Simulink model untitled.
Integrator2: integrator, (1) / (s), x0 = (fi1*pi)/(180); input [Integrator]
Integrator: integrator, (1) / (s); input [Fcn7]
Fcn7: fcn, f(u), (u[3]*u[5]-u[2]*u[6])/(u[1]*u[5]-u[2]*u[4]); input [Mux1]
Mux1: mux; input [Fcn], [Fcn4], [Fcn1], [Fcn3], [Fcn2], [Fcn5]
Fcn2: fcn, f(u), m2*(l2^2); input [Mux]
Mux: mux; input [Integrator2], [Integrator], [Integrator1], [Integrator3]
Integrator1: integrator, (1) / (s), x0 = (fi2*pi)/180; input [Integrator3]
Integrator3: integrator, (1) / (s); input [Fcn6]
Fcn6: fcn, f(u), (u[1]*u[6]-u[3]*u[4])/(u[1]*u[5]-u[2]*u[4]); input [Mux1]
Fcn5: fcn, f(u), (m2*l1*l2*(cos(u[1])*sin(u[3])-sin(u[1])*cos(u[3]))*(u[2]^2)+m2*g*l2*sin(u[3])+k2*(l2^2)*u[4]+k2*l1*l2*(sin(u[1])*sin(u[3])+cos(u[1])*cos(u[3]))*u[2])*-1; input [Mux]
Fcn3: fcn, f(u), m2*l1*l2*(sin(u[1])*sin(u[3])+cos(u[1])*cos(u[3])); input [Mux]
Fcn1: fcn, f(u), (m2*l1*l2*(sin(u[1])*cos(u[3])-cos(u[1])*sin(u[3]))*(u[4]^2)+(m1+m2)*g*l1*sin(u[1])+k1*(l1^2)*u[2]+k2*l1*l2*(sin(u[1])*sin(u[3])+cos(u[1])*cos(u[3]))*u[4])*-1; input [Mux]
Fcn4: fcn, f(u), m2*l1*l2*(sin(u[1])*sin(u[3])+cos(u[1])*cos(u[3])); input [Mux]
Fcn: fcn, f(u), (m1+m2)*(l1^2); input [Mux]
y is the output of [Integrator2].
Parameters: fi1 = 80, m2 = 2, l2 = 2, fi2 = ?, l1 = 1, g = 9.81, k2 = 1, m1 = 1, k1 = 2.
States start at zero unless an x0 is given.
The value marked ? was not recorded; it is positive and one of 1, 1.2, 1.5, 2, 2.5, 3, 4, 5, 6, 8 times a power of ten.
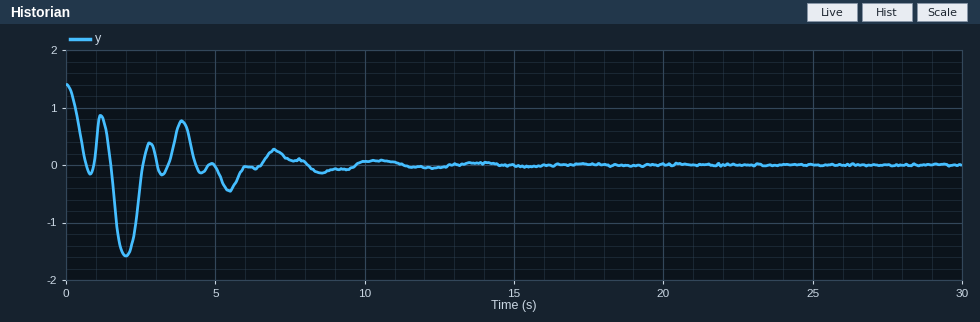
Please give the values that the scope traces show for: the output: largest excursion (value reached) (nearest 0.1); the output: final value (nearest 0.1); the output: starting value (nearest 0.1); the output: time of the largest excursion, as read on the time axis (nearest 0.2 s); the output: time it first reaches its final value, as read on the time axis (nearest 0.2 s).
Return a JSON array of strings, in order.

["-1.6", "0.0", "1.4", "2.0 s", "0.6 s"]
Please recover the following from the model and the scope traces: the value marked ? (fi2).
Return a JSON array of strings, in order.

["150"]
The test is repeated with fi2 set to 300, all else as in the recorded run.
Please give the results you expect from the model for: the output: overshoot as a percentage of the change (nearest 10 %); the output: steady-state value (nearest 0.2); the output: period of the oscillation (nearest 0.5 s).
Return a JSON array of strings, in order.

["80 %", "0.0", "1.5 s"]
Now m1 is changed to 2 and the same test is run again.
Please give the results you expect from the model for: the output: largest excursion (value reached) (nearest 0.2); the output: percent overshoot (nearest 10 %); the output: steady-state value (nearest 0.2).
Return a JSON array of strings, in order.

["-1.2", "90 %", "0.0"]
